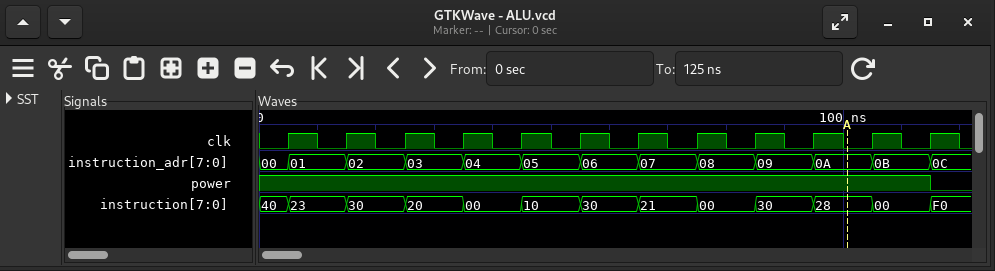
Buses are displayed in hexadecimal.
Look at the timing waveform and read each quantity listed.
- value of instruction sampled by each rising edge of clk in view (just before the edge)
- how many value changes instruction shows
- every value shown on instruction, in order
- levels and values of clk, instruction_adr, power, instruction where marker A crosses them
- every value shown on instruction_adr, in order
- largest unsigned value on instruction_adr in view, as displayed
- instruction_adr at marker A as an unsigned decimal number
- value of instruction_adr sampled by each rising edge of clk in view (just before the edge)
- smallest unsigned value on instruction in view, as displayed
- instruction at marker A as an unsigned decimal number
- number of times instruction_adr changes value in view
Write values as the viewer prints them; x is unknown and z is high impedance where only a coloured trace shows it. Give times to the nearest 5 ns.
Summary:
40, 23, 30, 20, 00, 10, 30, 21, 00, 30, 28, 00
12
40, 23, 30, 20, 00, 10, 30, 21, 00, 30, 28, 00, F0
clk=0, instruction_adr=0A, power=1, instruction=28
00, 01, 02, 03, 04, 05, 06, 07, 08, 09, 0A, 0B, 0C
0C
10
00, 01, 02, 03, 04, 05, 06, 07, 08, 09, 0A, 0B
00
40
12
